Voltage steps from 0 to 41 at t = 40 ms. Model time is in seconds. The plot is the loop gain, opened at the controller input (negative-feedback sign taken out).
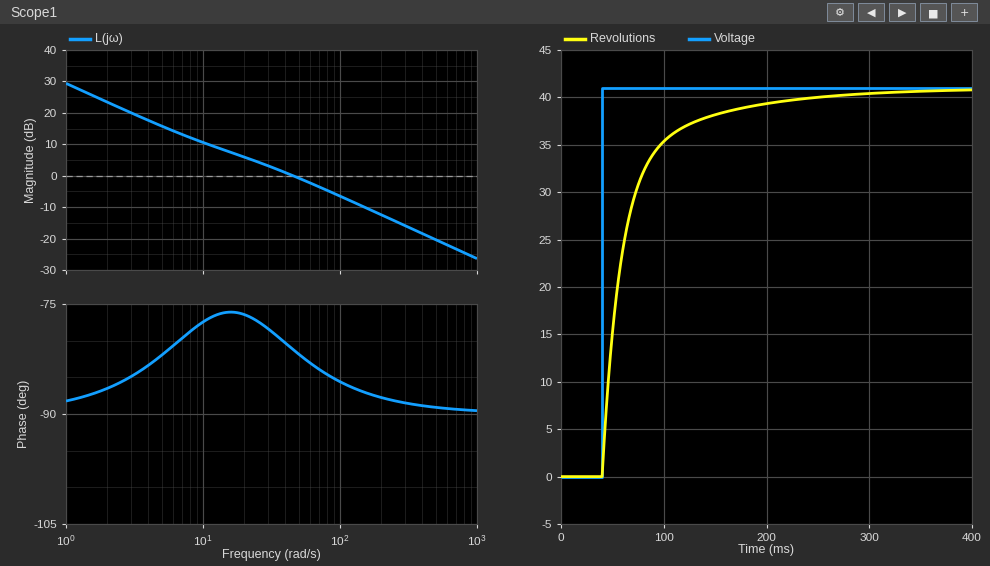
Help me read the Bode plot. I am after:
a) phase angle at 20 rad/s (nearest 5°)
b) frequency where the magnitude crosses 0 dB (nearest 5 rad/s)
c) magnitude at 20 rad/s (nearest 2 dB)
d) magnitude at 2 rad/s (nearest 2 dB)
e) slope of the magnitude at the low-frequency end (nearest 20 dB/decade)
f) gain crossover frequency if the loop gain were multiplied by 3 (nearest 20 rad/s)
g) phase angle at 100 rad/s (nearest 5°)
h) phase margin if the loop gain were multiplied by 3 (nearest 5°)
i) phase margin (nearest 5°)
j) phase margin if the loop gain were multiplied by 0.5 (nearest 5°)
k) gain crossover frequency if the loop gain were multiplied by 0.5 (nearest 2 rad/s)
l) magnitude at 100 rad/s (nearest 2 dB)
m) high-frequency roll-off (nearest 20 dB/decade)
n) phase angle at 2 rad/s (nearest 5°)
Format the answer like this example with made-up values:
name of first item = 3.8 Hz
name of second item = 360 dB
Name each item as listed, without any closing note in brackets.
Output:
phase angle at 20 rad/s = -75°
frequency where the magnitude crosses 0 dB = 45 rad/s
magnitude at 20 rad/s = 6 dB
magnitude at 2 rad/s = 24 dB
slope of the magnitude at the low-frequency end = -20 dB/decade
gain crossover frequency if the loop gain were multiplied by 3 = 140 rad/s
phase angle at 100 rad/s = -85°
phase margin if the loop gain were multiplied by 3 = 95°
phase margin = 100°
phase margin if the loop gain were multiplied by 0.5 = 105°
gain crossover frequency if the loop gain were multiplied by 0.5 = 20 rad/s
magnitude at 100 rad/s = -6 dB
high-frequency roll-off = -20 dB/decade
phase angle at 2 rad/s = -85°
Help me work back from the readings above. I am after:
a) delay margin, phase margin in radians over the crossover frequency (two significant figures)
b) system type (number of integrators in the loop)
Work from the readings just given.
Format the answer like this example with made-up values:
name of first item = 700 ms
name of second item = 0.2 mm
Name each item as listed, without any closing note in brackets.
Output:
delay margin, phase margin in radians over the crossover frequency = 0.039 s
system type = 1
